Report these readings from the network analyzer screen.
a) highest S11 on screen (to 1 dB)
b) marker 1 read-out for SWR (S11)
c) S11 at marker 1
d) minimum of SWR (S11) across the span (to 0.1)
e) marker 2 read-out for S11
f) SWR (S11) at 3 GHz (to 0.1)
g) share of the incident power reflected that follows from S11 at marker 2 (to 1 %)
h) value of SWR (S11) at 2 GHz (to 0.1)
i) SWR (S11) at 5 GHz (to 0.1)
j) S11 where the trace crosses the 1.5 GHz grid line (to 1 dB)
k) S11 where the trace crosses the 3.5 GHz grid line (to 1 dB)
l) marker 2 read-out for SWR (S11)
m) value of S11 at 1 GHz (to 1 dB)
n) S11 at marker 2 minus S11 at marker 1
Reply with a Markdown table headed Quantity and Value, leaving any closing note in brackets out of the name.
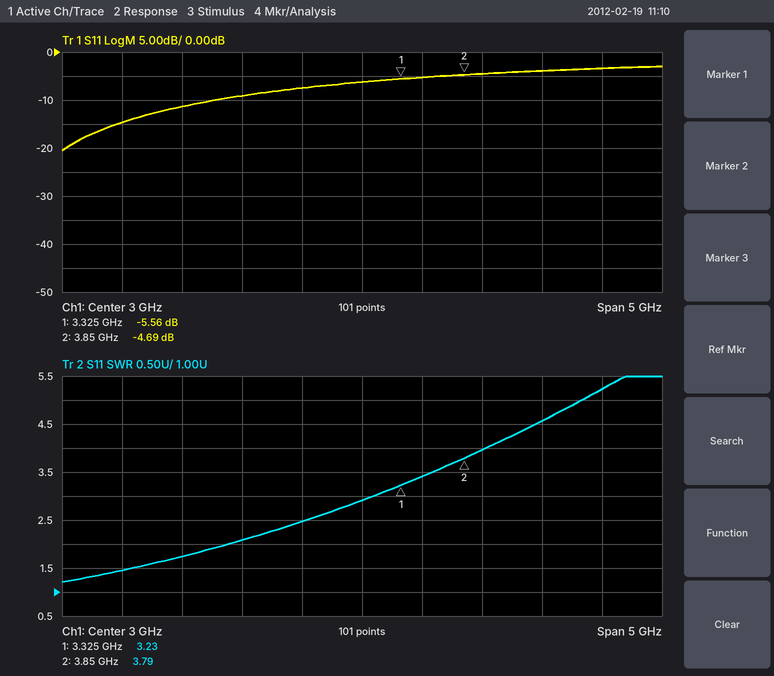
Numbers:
| Quantity | Value |
|---|---|
| highest S11 on screen | -3 dB |
| marker 1 read-out for SWR | 3.23 |
| S11 at marker 1 | -5.56 dB |
| minimum of SWR (S11) across the span | 1.2 |
| marker 2 read-out for S11 | -4.69 dB |
| SWR (S11) at 3 GHz | 2.9 |
| share of the incident power reflected that follows from S11 at marker 2 | 34 % |
| value of SWR (S11) at 2 GHz | 2.1 |
| SWR (S11) at 5 GHz | 5.2 |
| S11 where the trace crosses the 1.5 GHz grid line | -11 dB |
| S11 where the trace crosses the 3.5 GHz grid line | -5 dB |
| marker 2 read-out for SWR | 3.79 |
| value of S11 at 1 GHz | -15 dB |
| S11 at marker 2 minus S11 at marker 1 | 0.87 dB |
